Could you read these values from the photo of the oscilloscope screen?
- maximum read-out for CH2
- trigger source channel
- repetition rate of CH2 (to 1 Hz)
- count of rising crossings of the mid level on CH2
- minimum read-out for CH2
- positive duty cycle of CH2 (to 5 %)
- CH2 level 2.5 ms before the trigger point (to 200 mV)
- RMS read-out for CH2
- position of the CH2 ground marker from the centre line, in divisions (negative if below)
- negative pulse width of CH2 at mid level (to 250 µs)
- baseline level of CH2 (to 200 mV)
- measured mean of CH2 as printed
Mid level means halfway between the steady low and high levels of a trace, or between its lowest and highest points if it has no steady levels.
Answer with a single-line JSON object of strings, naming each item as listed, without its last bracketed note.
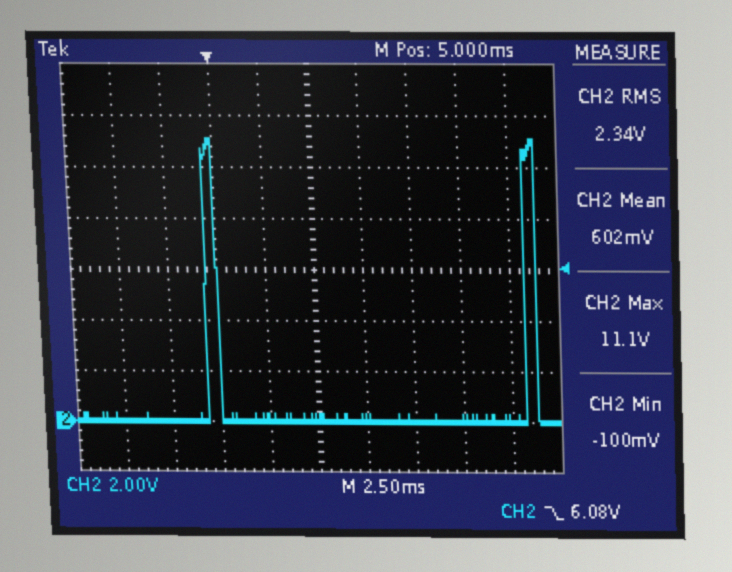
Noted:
{"maximum read-out for CH2": "11.1 V", "trigger source channel": "CH2", "repetition rate of CH2": "61 Hz", "count of rising crossings of the mid level on CH2": "2", "minimum read-out for CH2": "-100 mV", "positive duty cycle of CH2": "5 %", "CH2 level 2.5 ms before the trigger point": "0.0 V", "RMS read-out for CH2": "2.34 V", "position of the CH2 ground marker from the centre line, in divisions": "-3.0 div", "negative pulse width of CH2 at mid level": "15.75 ms", "baseline level of CH2": "0.0 V", "measured mean of CH2 as printed": "602 mV"}
